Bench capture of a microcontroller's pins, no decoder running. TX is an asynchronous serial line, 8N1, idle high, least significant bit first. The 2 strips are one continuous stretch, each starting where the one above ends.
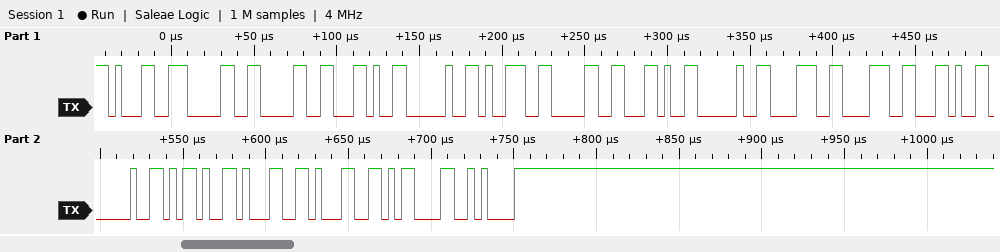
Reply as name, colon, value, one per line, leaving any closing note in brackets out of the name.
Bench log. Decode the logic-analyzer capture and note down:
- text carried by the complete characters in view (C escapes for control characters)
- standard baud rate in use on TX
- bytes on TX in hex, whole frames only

text carried by the complete characters in view: "100, 90, 88, -11\r\n"
standard baud rate in use on TX: 250000 baud
bytes on TX in hex, whole frames only: 0x31 0x30 0x30 0x2C 0x20 0x39 0x30 0x2C 0x20 0x38 0x38 0x2C 0x20 0x2D 0x31 0x31 0x0D 0x0A
